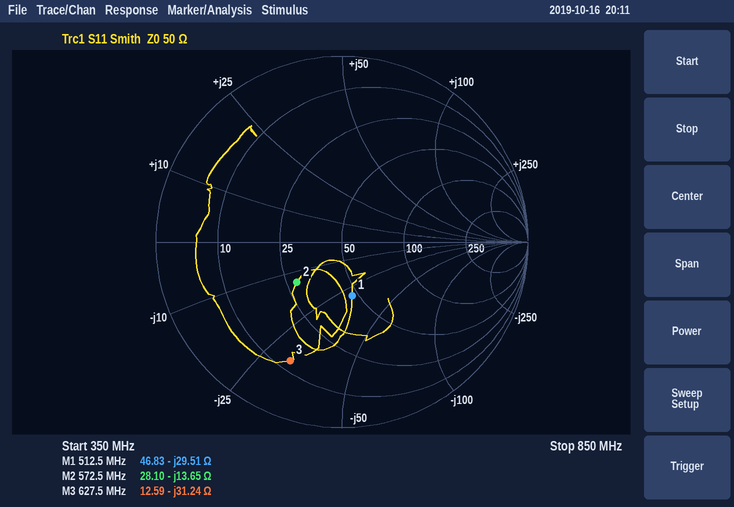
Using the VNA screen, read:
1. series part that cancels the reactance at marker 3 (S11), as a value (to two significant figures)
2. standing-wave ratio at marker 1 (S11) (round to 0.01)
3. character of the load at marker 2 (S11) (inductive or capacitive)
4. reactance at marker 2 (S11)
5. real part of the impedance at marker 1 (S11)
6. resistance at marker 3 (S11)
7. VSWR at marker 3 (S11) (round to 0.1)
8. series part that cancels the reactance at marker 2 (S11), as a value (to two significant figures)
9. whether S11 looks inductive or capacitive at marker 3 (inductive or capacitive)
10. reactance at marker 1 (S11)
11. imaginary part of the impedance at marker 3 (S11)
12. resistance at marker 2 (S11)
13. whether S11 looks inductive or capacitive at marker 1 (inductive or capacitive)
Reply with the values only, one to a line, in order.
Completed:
7.9 nH
1.83
capacitive
-13.65 Ω
46.83 Ω
12.59 Ω
5.6
3.8 nH
capacitive
-29.51 Ω
-31.24 Ω
28.10 Ω
capacitive
